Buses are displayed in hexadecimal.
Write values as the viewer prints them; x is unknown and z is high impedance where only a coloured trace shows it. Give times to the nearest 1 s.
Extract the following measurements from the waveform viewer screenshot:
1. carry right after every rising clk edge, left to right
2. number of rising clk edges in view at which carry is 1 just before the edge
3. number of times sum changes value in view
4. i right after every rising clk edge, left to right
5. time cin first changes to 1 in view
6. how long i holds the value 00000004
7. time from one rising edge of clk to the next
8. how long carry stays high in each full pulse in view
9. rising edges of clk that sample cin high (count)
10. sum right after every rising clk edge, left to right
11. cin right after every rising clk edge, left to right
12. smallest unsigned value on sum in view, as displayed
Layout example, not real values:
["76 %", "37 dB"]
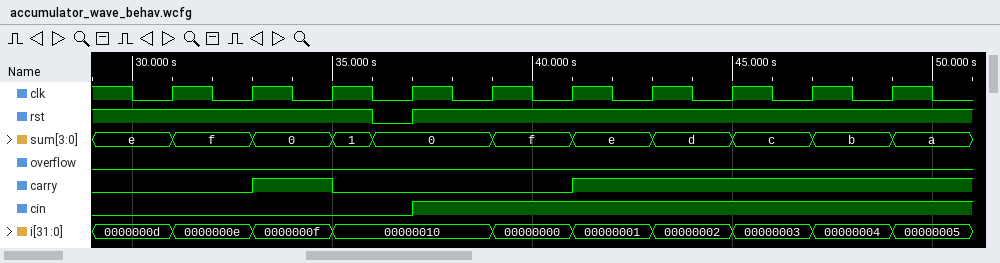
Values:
["0 1 0 0 0 1 1 1 1 1", "5", "10", "0000000e, 0000000f, 00000010, 00000010, 00000000, 00000001, 00000002, 00000003, 00000004, 00000005", "37 s", "2 s", "2 s", "2 s", "6", "f, 0, 1, 0, f, e, d, c, b, a", "0 0 0 1 1 1 1 1 1 1", "0"]
